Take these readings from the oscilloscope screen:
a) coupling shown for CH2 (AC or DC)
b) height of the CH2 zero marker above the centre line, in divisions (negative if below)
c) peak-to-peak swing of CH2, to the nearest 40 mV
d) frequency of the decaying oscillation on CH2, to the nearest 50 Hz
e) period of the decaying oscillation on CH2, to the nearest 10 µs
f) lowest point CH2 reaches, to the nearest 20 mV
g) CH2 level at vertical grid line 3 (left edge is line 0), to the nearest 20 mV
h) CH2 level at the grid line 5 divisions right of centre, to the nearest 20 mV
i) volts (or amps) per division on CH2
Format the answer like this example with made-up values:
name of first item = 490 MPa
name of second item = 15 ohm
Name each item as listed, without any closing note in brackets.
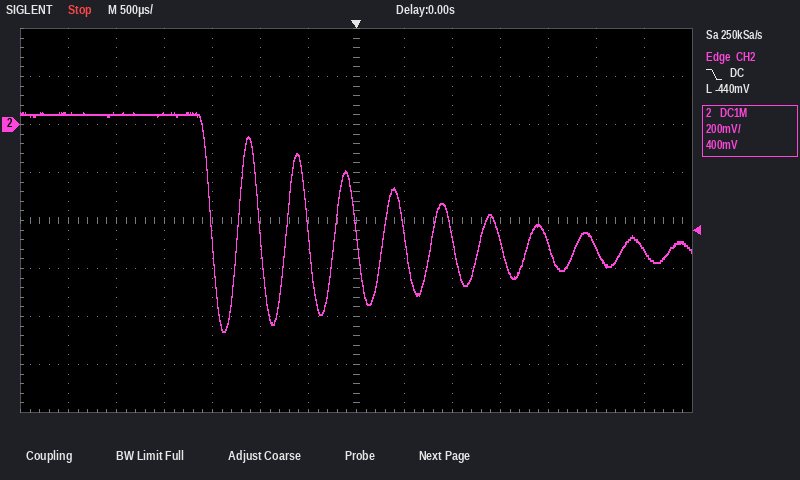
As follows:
coupling shown for CH2 = DC
height of the CH2 zero marker above the centre line, in divisions = +2.0 div
peak-to-peak swing of CH2, to the nearest 40 mV = 920 mV
frequency of the decaying oscillation on CH2, to the nearest 50 Hz = 2.00 kHz
period of the decaying oscillation on CH2, to the nearest 10 µs = 500 µs
lowest point CH2 reaches, to the nearest 20 mV = -860 mV
CH2 level at vertical grid line 3 (left edge is line 0), to the nearest 20 mV = 40 mV
CH2 level at the grid line 5 divisions right of centre, to the nearest 20 mV = -520 mV
volts (or amps) per division on CH2 = 200 mV
